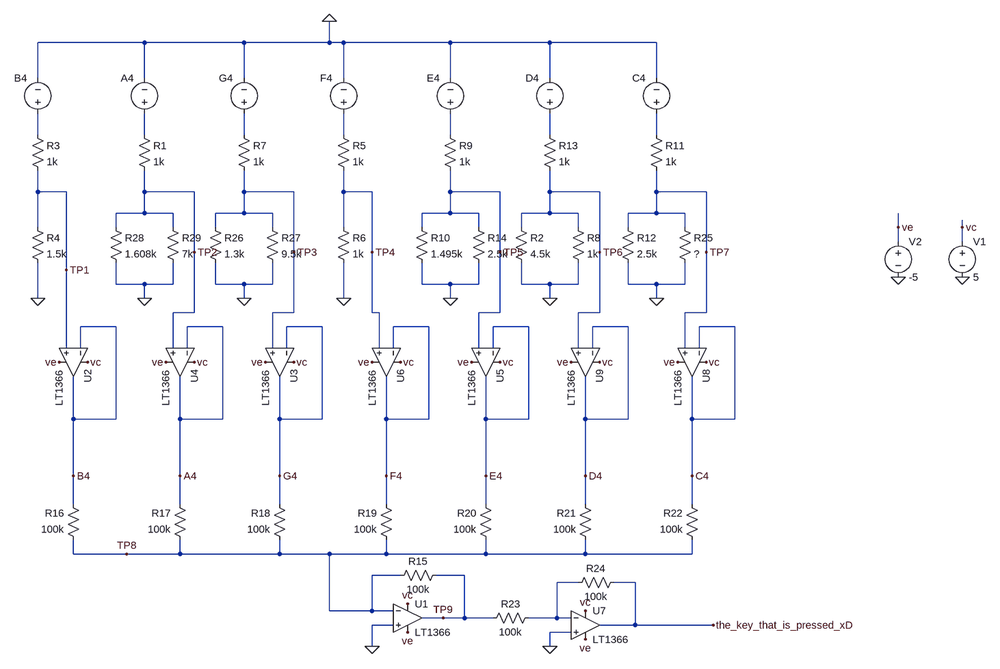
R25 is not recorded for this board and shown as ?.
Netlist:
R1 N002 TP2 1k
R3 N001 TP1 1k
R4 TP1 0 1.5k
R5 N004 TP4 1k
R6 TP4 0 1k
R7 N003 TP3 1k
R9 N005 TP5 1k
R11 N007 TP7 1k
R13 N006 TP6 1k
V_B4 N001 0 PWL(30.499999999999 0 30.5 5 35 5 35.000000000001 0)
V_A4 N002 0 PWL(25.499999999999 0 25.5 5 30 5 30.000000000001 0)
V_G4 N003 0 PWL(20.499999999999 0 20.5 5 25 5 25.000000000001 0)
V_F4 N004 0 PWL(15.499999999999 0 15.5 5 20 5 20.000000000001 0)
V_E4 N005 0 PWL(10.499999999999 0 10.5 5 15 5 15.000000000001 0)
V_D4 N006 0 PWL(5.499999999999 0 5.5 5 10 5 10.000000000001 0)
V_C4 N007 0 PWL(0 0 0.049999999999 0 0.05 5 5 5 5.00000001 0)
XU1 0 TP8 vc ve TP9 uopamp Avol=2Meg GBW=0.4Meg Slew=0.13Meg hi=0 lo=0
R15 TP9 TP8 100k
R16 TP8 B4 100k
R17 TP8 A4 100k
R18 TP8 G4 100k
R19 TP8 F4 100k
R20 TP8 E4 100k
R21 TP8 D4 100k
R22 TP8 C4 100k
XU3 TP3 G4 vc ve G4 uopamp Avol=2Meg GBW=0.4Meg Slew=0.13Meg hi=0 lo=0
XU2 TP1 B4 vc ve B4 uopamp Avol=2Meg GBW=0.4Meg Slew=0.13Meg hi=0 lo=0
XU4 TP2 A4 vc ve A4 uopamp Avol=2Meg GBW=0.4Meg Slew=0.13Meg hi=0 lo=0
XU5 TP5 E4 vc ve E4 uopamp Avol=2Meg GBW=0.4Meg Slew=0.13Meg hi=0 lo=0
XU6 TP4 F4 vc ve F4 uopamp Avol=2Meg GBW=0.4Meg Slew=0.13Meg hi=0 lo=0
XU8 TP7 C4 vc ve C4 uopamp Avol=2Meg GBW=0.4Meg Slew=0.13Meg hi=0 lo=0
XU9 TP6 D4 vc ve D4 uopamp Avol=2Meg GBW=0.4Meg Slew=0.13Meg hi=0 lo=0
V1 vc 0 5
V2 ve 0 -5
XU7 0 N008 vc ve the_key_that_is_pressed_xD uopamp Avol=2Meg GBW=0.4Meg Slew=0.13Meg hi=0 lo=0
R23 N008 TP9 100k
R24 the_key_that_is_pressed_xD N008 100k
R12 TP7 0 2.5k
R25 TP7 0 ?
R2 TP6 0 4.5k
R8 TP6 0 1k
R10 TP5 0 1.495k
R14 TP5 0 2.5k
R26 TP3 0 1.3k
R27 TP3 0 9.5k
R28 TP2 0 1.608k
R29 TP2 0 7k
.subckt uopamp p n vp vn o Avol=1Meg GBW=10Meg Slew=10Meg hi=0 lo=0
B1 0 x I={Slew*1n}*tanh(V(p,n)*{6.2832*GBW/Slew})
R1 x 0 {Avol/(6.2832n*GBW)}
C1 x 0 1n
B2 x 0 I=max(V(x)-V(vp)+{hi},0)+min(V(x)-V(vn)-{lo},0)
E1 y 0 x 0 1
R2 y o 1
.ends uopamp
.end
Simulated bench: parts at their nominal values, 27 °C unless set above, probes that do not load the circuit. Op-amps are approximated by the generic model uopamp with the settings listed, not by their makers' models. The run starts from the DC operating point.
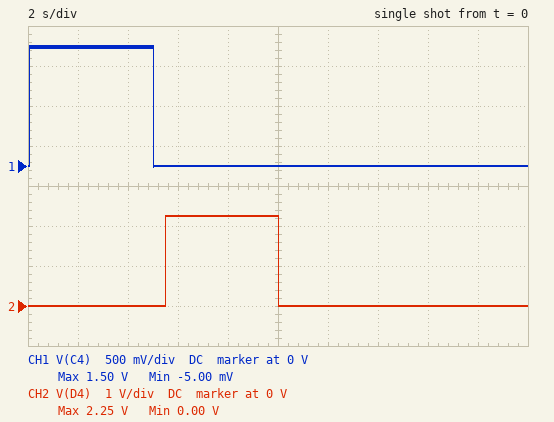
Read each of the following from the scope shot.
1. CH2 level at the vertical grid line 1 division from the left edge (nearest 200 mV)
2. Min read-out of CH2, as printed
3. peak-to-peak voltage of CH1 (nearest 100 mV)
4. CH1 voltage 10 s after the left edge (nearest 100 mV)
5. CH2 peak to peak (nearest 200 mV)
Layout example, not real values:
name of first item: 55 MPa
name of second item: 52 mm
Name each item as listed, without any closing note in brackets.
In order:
CH2 level at the vertical grid line 1 division from the left edge: 0 V
Min read-out of CH2, as printed: 0.00 V
peak-to-peak voltage of CH1: 1.5 V
CH1 voltage 10 s after the left edge: 0 V
CH2 peak to peak: 2.2 V
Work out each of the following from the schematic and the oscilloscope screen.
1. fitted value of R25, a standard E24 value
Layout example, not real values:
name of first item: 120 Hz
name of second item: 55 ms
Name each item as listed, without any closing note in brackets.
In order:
fitted value of R25, a standard E24 value: 510 Ω
